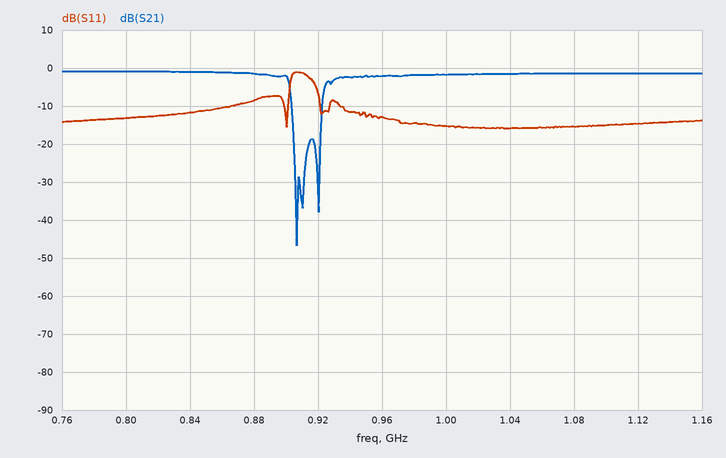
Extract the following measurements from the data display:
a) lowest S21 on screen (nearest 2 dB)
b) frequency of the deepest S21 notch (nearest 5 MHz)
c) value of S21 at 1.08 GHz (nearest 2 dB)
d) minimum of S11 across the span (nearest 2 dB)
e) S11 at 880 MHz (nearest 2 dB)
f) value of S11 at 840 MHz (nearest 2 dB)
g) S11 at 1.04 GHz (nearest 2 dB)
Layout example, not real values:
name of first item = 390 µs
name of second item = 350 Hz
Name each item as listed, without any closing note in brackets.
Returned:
lowest S21 on screen = -46 dB
frequency of the deepest S21 notch = 905 MHz
value of S21 at 1.08 GHz = -2 dB
minimum of S11 across the span = -16 dB
S11 at 880 MHz = -8 dB
value of S11 at 840 MHz = -12 dB
S11 at 1.04 GHz = -16 dB
